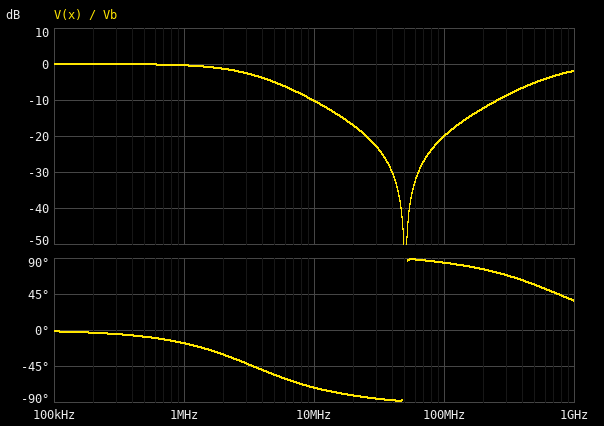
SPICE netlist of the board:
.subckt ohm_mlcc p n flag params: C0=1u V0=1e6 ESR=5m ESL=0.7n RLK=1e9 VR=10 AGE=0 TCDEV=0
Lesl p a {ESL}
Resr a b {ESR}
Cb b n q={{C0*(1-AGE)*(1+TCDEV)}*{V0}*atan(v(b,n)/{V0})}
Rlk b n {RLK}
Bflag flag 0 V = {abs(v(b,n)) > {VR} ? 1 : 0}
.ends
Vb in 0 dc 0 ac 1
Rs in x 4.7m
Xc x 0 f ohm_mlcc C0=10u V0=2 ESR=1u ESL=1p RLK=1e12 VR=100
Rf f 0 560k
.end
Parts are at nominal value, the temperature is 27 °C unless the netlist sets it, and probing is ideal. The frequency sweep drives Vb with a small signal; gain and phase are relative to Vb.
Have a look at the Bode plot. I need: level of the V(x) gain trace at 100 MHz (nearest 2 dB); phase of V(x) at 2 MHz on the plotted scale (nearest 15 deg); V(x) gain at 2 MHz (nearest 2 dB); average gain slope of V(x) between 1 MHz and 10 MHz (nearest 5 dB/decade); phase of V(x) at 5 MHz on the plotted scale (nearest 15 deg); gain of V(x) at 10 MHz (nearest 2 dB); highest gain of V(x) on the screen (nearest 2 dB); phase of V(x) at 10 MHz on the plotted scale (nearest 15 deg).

-20 dB
-30 deg
-2 dB
-10 dB/decade
-60 deg
-10 dB
0 dB
-75 deg
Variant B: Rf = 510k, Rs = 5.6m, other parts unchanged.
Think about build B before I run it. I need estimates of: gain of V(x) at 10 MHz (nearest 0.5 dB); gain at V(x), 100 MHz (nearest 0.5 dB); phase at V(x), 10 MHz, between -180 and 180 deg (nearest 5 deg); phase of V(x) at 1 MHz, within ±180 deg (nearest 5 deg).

-11.5 dB
-21.5 dB
-75 deg
-20 deg
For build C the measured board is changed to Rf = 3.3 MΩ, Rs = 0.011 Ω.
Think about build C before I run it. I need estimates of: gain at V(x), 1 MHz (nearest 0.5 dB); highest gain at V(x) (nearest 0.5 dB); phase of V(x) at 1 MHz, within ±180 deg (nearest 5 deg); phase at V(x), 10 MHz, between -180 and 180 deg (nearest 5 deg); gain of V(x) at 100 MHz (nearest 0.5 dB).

-1.5 dB
0 dB
-35 deg
-80 deg
-27.5 dB
